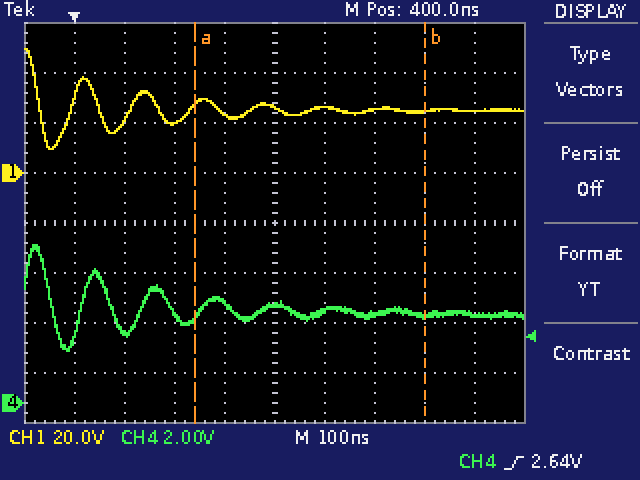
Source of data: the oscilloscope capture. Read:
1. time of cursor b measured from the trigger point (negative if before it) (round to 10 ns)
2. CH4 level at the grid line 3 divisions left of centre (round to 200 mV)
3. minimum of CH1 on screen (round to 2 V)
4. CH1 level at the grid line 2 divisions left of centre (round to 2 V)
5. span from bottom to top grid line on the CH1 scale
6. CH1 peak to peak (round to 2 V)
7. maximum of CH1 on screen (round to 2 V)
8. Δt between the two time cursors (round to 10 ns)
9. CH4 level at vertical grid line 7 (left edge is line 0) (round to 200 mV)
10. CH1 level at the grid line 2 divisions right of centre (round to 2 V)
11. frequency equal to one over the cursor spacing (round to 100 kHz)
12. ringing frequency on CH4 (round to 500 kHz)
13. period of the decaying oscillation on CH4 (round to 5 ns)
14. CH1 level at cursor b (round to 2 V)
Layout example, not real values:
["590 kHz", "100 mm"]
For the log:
["+700 ns", "2.8 V", "10 V", "20 V", "160 V", "40 V", "50 V", "460 ns", "3.6 V", "26 V", "2.2 MHz", "8.0 MHz", "125 ns", "24 V"]
